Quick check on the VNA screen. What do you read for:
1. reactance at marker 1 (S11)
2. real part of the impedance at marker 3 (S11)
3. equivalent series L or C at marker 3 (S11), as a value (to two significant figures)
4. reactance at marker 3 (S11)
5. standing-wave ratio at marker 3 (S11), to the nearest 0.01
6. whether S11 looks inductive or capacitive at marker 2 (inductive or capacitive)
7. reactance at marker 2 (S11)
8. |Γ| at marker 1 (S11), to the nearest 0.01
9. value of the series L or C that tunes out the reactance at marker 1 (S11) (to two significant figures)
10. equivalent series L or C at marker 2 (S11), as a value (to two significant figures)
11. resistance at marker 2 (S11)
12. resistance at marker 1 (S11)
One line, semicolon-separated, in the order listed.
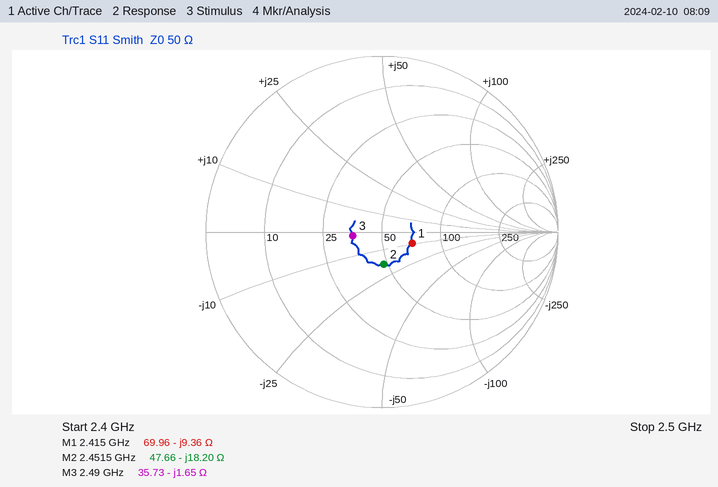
-9.36 Ω; 35.73 Ω; 39 pF; -1.65 Ω; 1.40; capacitive; -18.20 Ω; 0.18; 620 pH; 3.6 pF; 47.66 Ω; 69.96 Ω
